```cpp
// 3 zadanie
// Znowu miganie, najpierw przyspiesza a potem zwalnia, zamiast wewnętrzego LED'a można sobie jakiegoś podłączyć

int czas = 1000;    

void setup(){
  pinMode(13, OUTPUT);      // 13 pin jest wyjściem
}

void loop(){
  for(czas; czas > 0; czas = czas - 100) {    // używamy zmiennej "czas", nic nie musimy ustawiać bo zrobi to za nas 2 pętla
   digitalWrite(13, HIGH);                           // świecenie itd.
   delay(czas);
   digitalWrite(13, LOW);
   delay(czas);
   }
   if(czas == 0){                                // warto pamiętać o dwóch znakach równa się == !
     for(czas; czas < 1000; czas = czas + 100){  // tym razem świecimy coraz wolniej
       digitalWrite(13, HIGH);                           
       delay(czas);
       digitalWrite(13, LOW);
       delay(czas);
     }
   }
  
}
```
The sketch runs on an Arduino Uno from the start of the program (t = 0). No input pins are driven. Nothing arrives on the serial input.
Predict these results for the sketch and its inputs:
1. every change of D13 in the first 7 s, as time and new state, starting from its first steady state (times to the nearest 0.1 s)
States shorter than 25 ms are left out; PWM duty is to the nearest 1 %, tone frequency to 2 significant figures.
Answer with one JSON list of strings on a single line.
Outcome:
["0 s high; 1 s low; 2 s high; 2.9 s low; 3.8 s high; 4.6 s low; 5.4 s high; 6.1 s low; 6.8 s high"]
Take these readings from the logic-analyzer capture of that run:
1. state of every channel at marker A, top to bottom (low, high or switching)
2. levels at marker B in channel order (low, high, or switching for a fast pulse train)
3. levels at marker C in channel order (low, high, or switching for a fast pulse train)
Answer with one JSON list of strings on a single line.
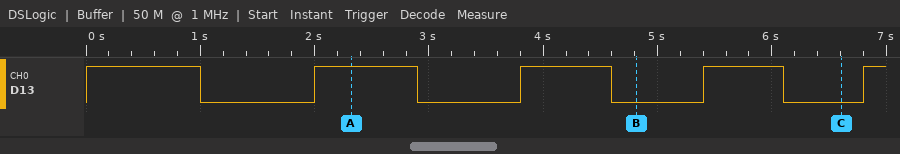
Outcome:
["D13 high", "D13 low", "D13 low"]
